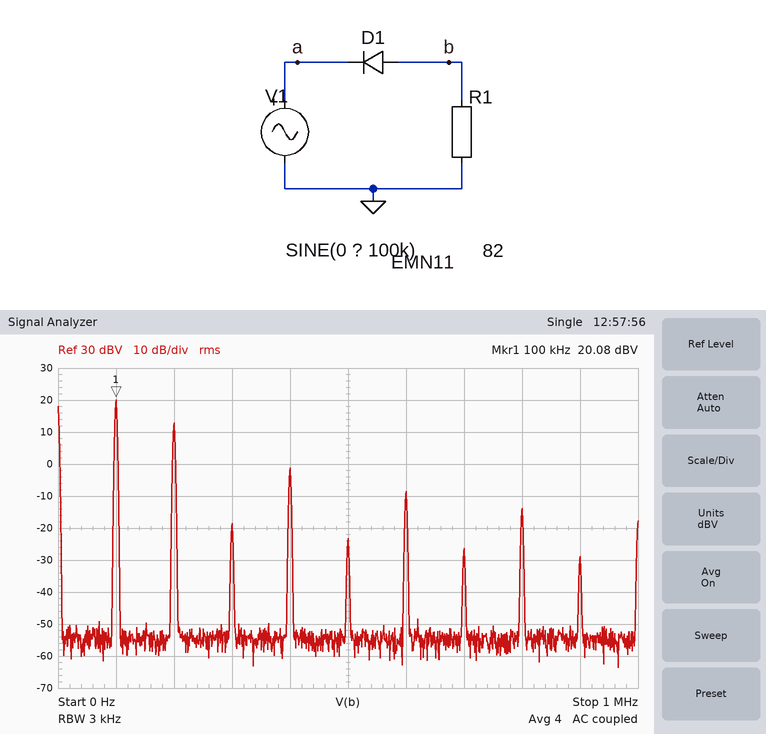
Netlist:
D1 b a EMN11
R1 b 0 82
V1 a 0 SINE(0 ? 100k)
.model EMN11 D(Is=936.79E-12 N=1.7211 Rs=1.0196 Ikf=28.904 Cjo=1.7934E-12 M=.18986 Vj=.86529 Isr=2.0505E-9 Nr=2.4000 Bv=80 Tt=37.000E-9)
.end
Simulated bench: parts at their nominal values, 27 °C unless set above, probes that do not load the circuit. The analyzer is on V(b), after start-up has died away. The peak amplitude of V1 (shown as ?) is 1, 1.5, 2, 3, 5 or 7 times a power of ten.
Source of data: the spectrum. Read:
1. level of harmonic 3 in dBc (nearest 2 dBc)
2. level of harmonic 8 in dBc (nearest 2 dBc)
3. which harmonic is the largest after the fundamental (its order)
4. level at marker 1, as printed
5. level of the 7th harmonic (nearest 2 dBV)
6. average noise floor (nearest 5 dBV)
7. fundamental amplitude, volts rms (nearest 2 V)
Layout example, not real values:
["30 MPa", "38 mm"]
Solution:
["-38 dBc", "-34 dBc", "2", "20.08 dBV", "-26 dBV", "-55 dBV", "10 V"]
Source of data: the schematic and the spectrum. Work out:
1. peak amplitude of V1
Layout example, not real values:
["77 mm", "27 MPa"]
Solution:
["30 V"]
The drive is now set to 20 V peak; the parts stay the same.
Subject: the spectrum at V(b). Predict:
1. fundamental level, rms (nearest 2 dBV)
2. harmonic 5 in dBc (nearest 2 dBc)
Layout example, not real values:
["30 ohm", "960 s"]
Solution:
["16 dBV", "-40 dBc"]
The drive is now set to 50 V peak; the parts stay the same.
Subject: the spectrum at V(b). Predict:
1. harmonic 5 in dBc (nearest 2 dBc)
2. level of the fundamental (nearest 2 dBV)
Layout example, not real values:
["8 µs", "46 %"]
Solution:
["-48 dBc", "24 dBV"]
